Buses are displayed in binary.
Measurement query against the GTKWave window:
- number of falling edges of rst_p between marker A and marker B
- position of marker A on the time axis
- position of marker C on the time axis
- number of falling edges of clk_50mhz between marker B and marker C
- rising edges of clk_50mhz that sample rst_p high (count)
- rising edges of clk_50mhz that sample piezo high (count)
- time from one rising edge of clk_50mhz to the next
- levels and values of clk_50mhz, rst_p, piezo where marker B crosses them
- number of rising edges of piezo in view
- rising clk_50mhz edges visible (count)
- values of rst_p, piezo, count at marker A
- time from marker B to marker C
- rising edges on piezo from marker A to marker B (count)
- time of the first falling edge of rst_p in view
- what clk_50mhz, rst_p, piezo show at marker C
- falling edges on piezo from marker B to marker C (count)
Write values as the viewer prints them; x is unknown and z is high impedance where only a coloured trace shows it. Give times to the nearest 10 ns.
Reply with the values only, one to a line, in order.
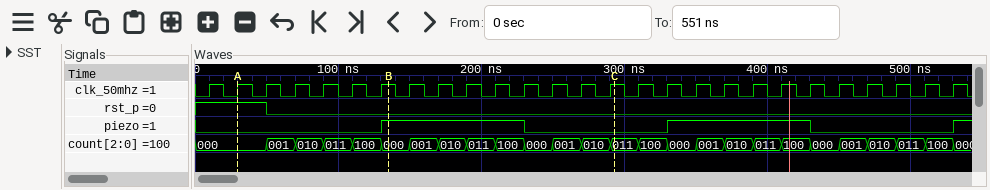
1
30 ns
290 ns
8
3
10
20 ns
clk_50mhz=1, rst_p=0, piezo=1
3
27
rst_p=1, piezo=0, count=000
160 ns
1
50 ns
clk_50mhz=1, rst_p=0, piezo=0
1
